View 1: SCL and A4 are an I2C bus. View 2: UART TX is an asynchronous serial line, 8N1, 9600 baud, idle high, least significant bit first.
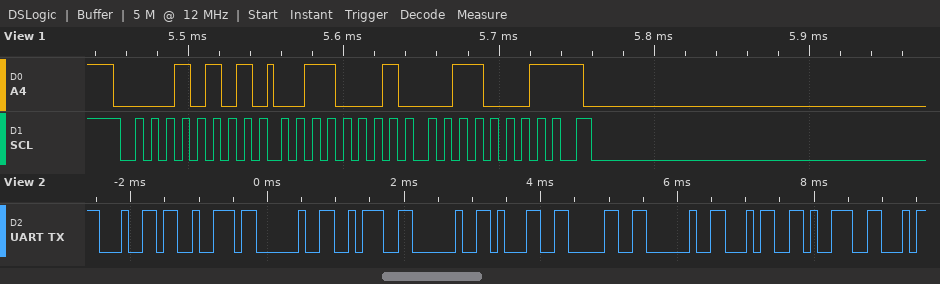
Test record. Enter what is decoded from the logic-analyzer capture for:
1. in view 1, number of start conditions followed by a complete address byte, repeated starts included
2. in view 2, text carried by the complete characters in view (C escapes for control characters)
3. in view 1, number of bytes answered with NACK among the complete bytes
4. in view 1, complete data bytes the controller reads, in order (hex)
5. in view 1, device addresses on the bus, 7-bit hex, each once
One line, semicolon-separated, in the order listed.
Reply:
1; "dr : 10 49"; 1; 31 31; 0x0A
